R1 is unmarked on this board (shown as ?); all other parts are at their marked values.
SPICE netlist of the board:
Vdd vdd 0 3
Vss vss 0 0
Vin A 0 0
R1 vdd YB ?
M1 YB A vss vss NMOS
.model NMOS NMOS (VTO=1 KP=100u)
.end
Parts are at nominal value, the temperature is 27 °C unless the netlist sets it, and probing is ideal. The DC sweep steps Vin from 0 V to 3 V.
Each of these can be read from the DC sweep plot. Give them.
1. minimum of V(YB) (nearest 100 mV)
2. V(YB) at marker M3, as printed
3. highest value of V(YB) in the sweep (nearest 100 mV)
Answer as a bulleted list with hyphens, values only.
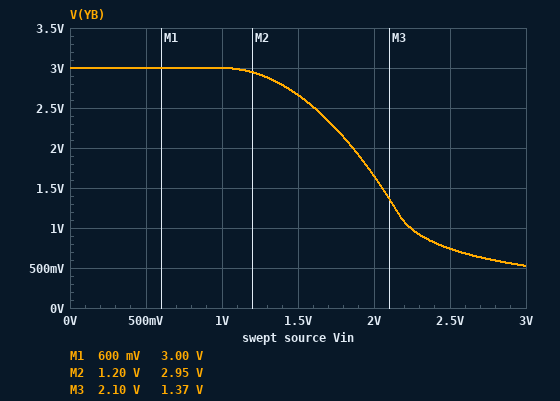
- 500 mV
- 1.37 V
- 3.0 V
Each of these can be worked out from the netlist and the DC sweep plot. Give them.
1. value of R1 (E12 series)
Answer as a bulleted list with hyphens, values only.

- 27 kΩ
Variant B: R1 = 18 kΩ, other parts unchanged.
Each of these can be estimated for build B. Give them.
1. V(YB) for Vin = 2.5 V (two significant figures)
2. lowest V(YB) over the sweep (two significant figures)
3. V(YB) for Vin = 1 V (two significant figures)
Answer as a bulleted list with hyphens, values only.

- 1.1 V
- 770 mV
- 3.0 V
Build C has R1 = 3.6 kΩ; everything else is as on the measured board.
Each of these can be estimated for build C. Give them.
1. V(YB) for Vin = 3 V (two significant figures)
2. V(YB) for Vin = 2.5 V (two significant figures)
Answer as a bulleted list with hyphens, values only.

- 2.3 V
- 2.6 V
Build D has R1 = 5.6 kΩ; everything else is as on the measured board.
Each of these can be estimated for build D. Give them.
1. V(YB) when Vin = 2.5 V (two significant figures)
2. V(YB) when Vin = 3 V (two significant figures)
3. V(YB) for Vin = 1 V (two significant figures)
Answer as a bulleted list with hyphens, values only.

- 2.4 V
- 1.9 V
- 3.0 V
